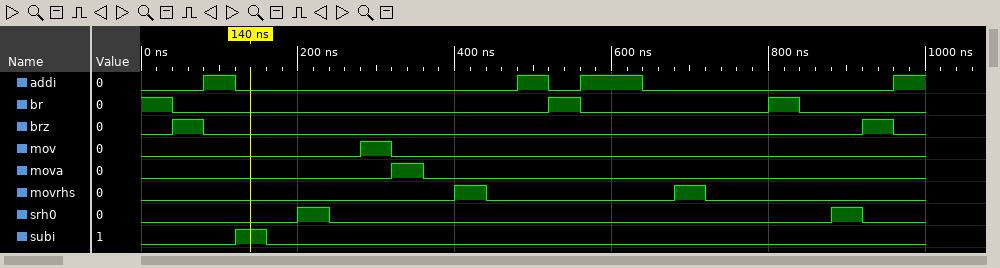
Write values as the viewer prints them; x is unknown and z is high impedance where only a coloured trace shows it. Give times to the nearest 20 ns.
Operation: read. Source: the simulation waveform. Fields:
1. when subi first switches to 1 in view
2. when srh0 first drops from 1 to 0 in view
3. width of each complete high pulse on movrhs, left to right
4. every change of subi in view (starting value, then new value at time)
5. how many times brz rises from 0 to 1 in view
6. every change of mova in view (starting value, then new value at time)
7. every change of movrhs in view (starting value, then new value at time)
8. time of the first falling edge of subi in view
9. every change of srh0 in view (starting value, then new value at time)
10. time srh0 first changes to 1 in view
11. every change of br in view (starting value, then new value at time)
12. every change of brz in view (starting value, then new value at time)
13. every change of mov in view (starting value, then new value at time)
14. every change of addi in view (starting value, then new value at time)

120 ns
240 ns
40 ns, 40 ns
0, 1 at 120 ns, 0 at 160 ns
2
0, 1 at 320 ns, 0 at 360 ns
0, 1 at 400 ns, 0 at 440 ns, 1 at 680 ns, 0 at 720 ns
160 ns
0, 1 at 200 ns, 0 at 240 ns, 1 at 880 ns, 0 at 920 ns
200 ns
1, 0 at 40 ns, 1 at 520 ns, 0 at 560 ns, 1 at 800 ns, 0 at 840 ns
0, 1 at 40 ns, 0 at 80 ns, 1 at 920 ns, 0 at 960 ns
0, 1 at 280 ns, 0 at 320 ns
0, 1 at 80 ns, 0 at 120 ns, 1 at 480 ns, 0 at 520 ns, 1 at 560 ns, 0 at 640 ns, 1 at 960 ns
